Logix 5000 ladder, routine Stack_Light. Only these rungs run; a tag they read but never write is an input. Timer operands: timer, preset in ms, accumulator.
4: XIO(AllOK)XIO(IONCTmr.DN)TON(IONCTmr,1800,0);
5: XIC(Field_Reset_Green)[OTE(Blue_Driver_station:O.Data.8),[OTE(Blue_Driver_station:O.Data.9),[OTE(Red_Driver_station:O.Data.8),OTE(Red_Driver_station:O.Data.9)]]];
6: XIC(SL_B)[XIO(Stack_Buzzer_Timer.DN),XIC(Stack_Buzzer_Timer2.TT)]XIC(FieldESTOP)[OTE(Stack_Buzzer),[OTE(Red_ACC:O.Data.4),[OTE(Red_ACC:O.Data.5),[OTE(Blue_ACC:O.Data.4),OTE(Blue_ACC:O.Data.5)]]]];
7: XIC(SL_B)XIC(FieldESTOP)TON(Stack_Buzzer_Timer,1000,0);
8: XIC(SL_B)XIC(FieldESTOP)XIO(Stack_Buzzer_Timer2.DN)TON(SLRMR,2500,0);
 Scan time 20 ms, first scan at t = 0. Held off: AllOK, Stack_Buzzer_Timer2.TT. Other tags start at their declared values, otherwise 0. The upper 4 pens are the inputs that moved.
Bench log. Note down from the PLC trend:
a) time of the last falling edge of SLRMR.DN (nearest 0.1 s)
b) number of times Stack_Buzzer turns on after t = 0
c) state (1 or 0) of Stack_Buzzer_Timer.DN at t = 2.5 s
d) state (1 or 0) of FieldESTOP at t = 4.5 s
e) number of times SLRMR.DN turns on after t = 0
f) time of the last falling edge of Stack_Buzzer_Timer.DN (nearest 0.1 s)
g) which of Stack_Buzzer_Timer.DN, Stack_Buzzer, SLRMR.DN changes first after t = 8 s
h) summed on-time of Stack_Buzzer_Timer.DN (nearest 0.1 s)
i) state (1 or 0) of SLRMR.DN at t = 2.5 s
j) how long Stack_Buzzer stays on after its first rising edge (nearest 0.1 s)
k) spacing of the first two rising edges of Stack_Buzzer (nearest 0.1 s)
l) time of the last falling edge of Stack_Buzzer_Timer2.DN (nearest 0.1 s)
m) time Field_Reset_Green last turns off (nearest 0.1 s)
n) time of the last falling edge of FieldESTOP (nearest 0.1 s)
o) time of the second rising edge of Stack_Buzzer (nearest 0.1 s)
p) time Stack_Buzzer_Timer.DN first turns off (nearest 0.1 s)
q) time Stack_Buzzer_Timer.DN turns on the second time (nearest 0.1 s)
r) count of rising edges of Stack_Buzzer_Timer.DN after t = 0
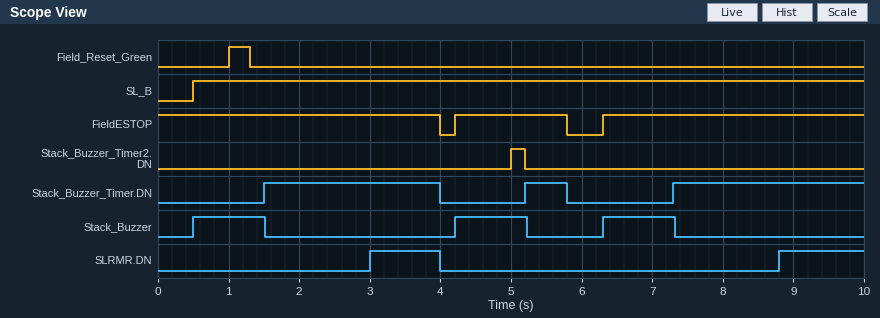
4.0 s
3
1
1
2
5.8 s
SLRMR.DN
5.8 s
0
1.0 s
3.7 s
5.2 s
1.3 s
5.8 s
4.2 s
4.0 s
5.2 s
3
